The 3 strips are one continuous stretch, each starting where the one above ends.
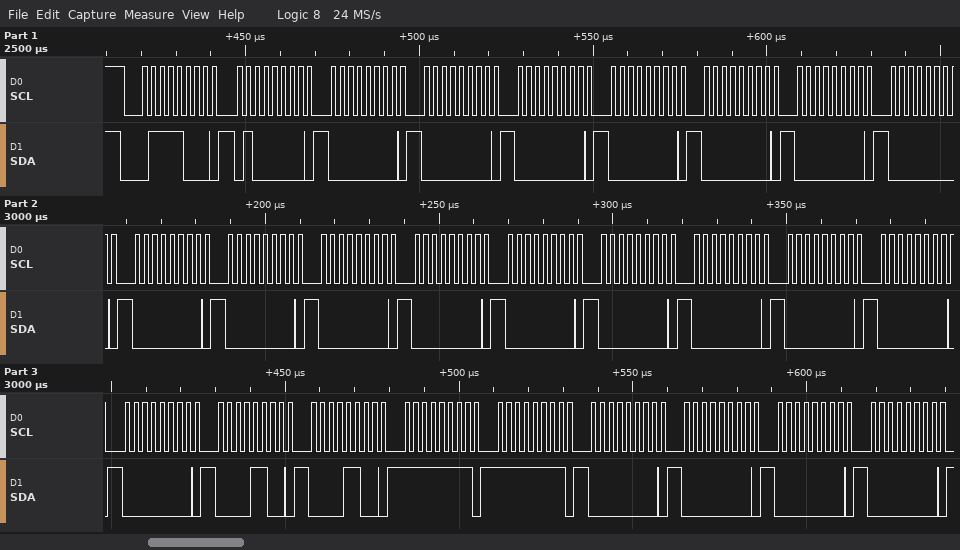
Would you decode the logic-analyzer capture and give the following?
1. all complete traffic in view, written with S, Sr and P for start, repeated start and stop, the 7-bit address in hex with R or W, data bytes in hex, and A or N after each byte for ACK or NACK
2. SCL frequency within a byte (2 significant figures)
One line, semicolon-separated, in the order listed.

S 3CW A 40 A 00 A 00 A 00 A 00 A 00 A 00 A 00 A 00 A 00 A 00 A 00 A 00 A 00 A 00 A 00 A 00 A 00 A 0C A 0C A FF A FF A 00 A 00 A 00 A 00 A; 400 kHz
